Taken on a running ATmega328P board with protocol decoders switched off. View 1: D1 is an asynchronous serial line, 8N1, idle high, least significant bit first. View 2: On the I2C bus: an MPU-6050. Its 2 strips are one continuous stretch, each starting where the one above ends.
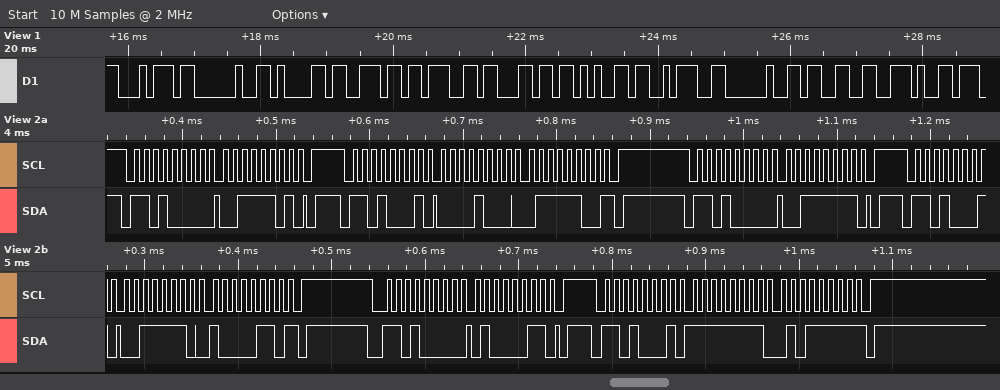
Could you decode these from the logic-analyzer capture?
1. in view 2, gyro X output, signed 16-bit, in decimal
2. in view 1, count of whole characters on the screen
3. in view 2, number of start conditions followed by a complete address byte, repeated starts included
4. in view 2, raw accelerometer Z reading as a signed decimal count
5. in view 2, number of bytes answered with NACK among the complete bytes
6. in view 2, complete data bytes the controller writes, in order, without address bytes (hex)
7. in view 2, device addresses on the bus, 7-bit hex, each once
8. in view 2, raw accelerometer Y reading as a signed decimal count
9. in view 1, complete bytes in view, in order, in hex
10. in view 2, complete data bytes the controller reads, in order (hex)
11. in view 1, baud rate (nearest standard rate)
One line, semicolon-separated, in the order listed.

-161; 11; 6; 16006; 3; 3D 3F 43; 0x68; 2172; 0x74 0x20 0x61 0x6E 0x67 0x6C 0x65 0x3A 0x20 0x33 0x2E; 08 7C 3E 86 FF 5F; 9600 baud
